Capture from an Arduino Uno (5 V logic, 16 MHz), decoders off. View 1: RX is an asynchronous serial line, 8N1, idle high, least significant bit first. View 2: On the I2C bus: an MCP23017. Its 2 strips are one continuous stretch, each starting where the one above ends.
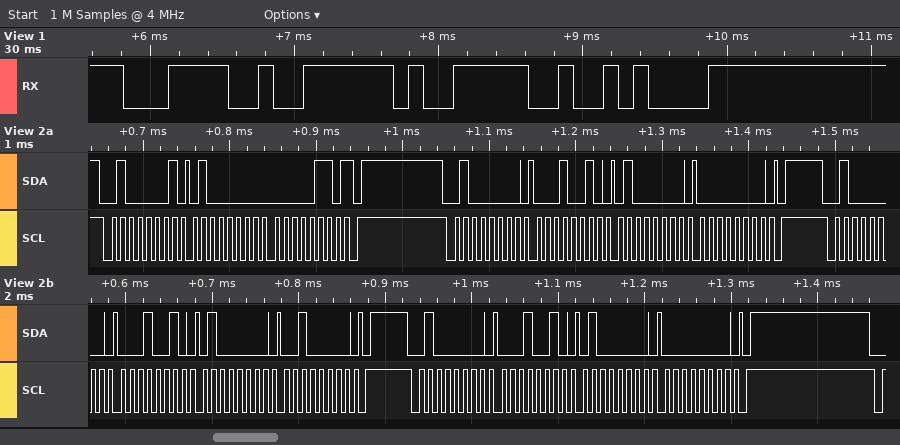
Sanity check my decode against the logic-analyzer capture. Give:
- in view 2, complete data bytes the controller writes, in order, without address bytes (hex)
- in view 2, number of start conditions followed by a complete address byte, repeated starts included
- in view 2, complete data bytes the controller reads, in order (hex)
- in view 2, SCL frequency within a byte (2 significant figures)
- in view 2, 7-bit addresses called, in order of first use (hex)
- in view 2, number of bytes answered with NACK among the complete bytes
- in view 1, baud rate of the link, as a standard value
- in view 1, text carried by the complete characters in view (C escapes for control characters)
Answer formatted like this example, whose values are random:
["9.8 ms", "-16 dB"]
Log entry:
["12 40 00 12 40 20 12 40 00", "4", "40 06", "100 kHz", "0x20", "1", "9600 baud", "\"<~>\\n\""]
